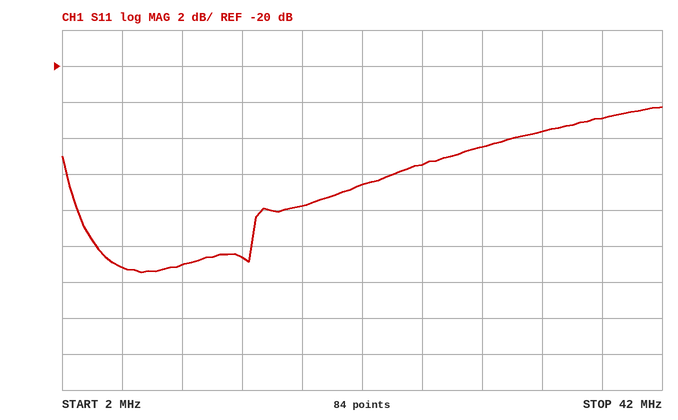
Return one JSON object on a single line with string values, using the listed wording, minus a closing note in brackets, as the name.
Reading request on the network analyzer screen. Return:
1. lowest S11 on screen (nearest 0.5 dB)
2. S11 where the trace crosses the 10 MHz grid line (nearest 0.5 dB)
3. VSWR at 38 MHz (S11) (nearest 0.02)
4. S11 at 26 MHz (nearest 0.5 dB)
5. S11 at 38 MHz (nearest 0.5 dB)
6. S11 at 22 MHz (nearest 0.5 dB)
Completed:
{"lowest S11 on screen": "-31.5 dB", "S11 where the trace crosses the 10 MHz grid line": "-31.0 dB", "VSWR at 38 MHz (S11)": "1.16", "S11 at 26 MHz": "-25.5 dB", "S11 at 38 MHz": "-23.0 dB", "S11 at 22 MHz": "-26.5 dB"}
